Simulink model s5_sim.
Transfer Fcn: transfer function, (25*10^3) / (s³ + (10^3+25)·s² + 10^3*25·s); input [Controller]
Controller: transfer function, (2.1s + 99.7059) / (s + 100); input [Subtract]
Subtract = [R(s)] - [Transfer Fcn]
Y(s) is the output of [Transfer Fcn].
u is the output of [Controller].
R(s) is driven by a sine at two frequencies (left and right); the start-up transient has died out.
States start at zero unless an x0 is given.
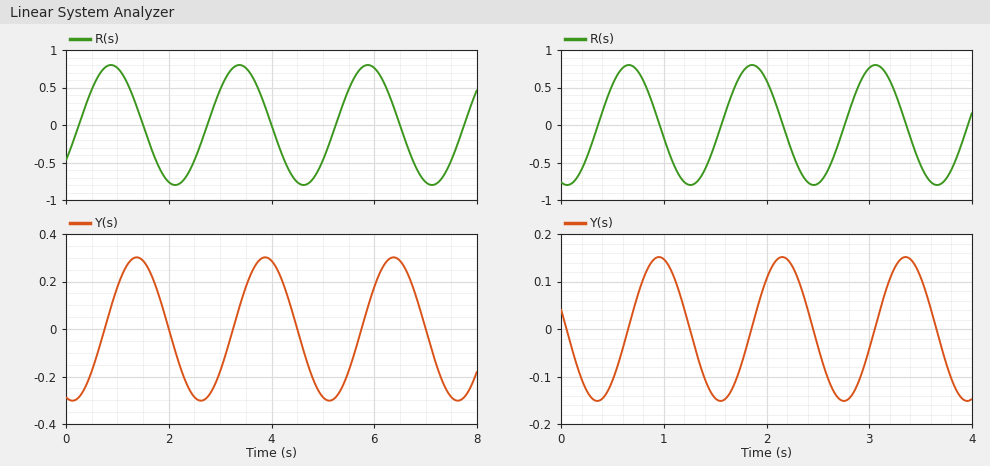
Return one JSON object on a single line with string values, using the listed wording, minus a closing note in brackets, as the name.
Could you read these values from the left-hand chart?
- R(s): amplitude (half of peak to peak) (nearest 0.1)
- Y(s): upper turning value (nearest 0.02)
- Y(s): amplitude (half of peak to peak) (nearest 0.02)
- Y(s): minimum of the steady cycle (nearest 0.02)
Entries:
{"R(s): amplitude (half of peak to peak)": "0.8", "Y(s): upper turning value": "0.30", "Y(s): amplitude (half of peak to peak)": "0.30", "Y(s): minimum of the steady cycle": "-0.30"}
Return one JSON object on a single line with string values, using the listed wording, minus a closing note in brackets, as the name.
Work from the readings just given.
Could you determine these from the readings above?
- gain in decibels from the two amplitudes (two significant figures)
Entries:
{"gain in decibels from the two amplitudes": "-8.5 dB"}
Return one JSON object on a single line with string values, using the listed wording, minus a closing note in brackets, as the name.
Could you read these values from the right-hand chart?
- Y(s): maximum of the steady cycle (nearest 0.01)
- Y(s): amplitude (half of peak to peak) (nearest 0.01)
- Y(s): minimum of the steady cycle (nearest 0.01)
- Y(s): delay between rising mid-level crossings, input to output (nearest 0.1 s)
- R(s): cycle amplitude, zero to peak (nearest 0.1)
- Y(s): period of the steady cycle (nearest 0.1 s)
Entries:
{"Y(s): maximum of the steady cycle": "0.15", "Y(s): amplitude (half of peak to peak)": "0.15", "Y(s): minimum of the steady cycle": "-0.15", "Y(s): delay between rising mid-level crossings, input to output": "0.3 s", "R(s): cycle amplitude, zero to peak": "0.8", "Y(s): period of the steady cycle": "1.2 s"}
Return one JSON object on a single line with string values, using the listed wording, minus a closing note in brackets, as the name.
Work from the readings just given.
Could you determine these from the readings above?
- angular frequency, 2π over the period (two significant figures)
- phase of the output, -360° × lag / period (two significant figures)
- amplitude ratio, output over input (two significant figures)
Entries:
{"angular frequency, 2π over the period": "5.2 rad/s", "phase of the output, -360° × lag / period": "-90°", "amplitude ratio, output over input": "0.19"}
